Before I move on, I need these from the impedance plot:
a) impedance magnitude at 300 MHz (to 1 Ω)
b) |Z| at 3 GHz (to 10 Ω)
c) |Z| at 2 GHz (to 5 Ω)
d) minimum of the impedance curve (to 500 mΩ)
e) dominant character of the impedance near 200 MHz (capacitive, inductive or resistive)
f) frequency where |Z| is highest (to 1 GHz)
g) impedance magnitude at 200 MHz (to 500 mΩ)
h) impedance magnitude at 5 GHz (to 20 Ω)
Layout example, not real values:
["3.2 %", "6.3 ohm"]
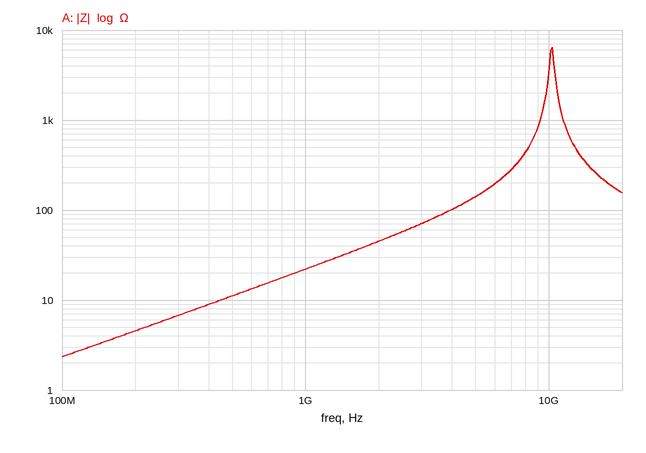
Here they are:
["7 Ω", "70 Ω", "45 Ω", "2.5 Ω", "inductive", "10 GHz", "4.5 Ω", "140 Ω"]
